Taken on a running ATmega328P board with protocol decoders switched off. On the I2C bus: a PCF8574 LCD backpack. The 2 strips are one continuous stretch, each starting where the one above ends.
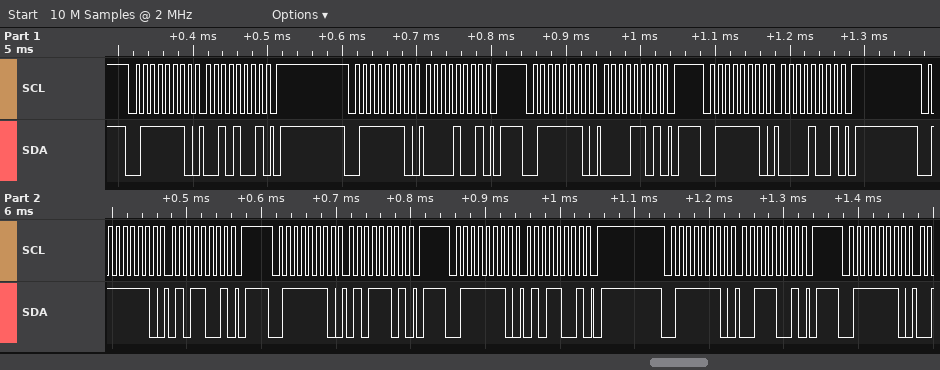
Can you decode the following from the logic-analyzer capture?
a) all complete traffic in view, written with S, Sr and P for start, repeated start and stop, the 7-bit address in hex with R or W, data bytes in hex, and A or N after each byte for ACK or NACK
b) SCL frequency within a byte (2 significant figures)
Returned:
S 3FW A 29 A P S 3FW A 09 A P S 3FW A 0D A P S 3FW A 09 A P S 3FW A 59 A P S 3FW A 5D A P S 3FW A 59 A P S 3FW A 39 A P S 3FW A
100 kHz
